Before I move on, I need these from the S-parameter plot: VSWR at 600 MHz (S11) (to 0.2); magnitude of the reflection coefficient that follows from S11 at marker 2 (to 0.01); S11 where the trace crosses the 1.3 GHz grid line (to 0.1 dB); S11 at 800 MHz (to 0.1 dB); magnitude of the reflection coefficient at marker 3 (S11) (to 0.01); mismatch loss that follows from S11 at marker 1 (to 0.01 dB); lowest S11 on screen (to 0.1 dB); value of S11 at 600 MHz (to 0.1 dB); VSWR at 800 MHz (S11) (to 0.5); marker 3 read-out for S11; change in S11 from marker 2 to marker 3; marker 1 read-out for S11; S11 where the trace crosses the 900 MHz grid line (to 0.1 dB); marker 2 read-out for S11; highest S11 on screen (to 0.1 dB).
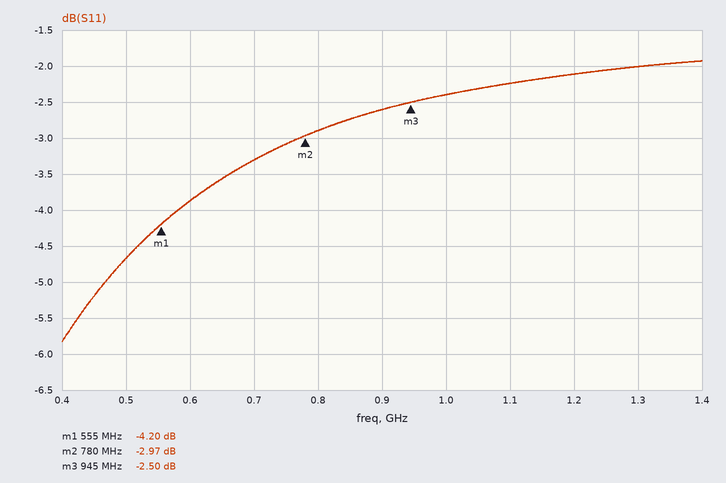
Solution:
4.6
0.71
-2.0 dB
-2.9 dB
0.75
2.08 dB
-5.8 dB
-3.9 dB
6.0
-2.50 dB
0.47 dB
-4.20 dB
-2.6 dB
-2.97 dB
-1.9 dB
